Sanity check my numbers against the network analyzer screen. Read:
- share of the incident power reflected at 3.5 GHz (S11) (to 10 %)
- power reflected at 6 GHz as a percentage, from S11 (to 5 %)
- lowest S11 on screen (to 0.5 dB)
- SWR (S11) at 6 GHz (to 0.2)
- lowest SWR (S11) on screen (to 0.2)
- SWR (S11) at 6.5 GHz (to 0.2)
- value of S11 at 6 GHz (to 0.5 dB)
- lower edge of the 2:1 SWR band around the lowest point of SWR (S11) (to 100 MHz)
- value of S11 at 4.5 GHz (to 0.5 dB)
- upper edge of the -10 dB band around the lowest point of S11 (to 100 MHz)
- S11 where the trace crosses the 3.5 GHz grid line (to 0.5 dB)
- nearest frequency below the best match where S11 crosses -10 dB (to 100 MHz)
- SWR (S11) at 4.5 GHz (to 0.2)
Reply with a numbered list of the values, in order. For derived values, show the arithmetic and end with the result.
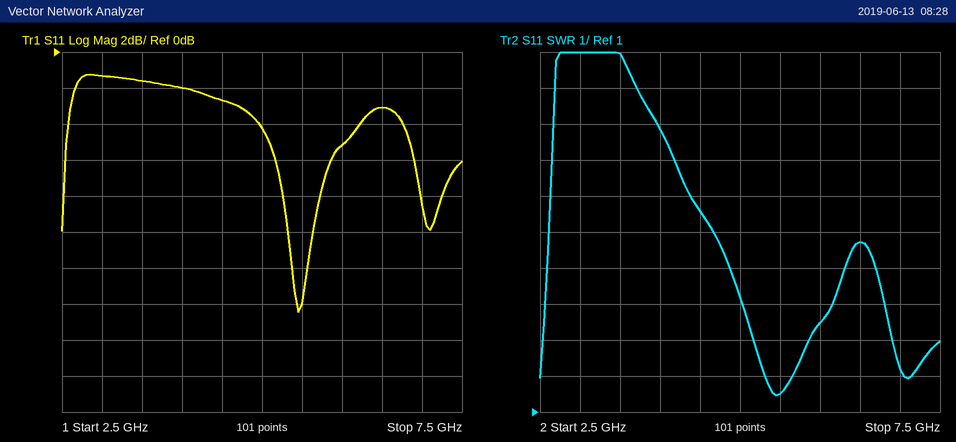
1. 10^(-1.5/10) ≈ 70.8 %, so 70 % to the nearest 10 %
2. 10^(-5/10) ≈ 31.6 %, so 30 % to the nearest 5 %
3. -14.5 dB
4. 3.4
5. 1.4
6. 5.8
7. -5.0 dB
8. 5.3 GHz
9. -2.5 dB
10. 5.6 GHz
11. -1.5 dB
12. 5.3 GHz
13. 6.6
